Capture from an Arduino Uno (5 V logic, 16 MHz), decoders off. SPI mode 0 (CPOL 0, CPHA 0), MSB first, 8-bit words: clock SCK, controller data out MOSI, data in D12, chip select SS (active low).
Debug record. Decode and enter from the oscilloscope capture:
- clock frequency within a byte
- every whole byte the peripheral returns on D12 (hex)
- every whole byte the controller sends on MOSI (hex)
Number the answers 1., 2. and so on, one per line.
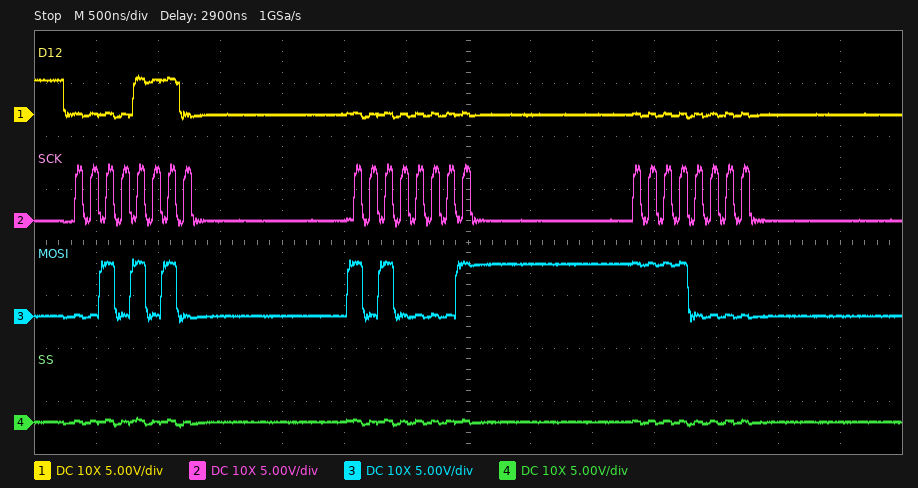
1. 8 MHz
2. 0E 00 00
3. 2A A1 F0
